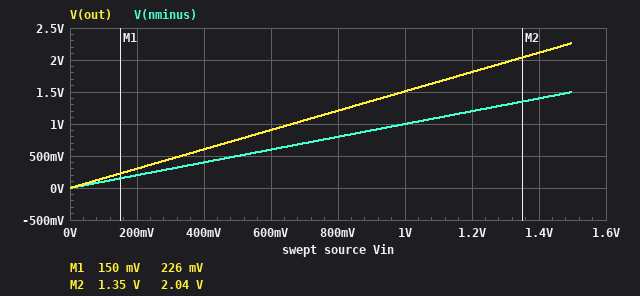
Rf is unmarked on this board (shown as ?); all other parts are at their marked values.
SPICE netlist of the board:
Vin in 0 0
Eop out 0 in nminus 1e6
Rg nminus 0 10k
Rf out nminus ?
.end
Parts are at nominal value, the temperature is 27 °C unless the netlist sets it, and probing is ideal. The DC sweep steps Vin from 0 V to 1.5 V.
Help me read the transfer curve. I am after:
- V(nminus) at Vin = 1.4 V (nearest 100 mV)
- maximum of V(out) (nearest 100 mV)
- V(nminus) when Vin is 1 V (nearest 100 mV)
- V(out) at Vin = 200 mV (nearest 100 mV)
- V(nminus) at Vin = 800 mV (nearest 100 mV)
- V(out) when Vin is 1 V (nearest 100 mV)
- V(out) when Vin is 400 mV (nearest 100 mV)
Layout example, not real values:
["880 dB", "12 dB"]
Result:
["1.4 V", "2.3 V", "1.0 V", "300 mV", "800 mV", "1.5 V", "600 mV"]
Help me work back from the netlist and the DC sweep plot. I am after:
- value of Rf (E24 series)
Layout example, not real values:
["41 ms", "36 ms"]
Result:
["5.1 kΩ"]
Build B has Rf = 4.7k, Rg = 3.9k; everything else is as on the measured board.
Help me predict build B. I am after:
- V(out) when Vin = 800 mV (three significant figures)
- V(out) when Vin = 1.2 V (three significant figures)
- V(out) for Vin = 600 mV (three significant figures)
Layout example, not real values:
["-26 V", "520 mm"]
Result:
["1.76 V", "2.65 V", "1.32 V"]
